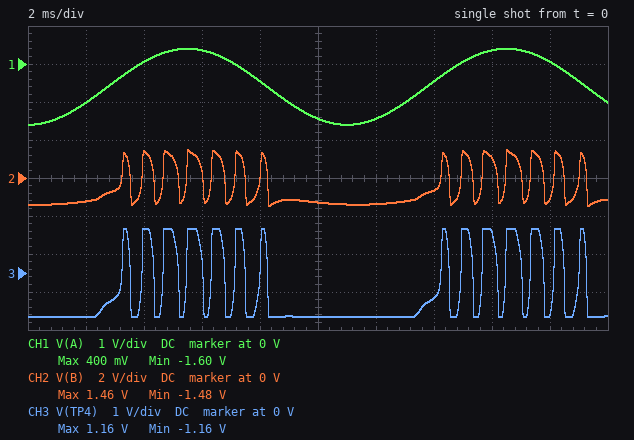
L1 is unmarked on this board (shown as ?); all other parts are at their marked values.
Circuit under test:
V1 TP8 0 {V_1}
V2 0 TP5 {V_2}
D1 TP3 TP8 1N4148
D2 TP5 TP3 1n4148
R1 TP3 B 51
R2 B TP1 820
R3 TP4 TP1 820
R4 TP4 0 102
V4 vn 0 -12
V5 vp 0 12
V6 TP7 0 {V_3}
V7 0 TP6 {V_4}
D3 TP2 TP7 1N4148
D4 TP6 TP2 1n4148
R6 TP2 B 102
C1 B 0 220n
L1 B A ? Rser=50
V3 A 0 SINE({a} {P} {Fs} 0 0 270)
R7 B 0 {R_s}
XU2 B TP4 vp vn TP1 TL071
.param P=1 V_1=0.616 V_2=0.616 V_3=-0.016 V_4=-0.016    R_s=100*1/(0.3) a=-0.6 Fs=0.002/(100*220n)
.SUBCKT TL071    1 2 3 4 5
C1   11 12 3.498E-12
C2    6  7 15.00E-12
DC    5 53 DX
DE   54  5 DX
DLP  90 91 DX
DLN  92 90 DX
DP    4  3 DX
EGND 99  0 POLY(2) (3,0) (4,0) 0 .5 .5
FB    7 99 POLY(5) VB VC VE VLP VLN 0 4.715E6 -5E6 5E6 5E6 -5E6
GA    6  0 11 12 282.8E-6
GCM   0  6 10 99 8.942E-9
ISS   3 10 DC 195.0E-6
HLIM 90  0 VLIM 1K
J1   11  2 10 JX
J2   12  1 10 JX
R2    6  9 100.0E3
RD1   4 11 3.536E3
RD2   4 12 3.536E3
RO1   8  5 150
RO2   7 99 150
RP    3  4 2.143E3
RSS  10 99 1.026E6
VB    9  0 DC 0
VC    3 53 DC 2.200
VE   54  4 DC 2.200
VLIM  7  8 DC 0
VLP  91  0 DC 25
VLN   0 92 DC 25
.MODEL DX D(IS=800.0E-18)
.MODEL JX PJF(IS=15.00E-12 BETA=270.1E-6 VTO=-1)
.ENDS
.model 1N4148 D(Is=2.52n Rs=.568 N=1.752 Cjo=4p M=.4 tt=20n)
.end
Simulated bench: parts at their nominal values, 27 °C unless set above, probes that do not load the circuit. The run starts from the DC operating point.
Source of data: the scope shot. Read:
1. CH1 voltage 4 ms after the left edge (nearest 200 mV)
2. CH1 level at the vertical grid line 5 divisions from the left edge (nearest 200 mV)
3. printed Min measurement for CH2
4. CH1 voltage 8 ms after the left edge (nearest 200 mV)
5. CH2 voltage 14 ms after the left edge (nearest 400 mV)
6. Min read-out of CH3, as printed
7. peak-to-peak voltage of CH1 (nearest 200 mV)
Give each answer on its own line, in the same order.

0 V
-1.4 V
-1.48 V
-400 mV
-800 mV
-1.16 V
2.0 V
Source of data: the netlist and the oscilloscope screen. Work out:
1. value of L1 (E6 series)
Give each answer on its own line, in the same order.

33 mH
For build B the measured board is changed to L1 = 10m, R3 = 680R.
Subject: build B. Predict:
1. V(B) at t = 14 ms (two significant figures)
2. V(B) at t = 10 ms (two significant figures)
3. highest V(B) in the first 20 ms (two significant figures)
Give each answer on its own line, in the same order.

-590 mV
-1.3 V
1.4 V
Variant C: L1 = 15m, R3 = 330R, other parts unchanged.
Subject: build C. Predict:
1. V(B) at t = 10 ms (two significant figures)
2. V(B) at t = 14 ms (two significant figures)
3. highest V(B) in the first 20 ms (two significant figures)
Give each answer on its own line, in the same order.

-1.2 V
-500 mV
430 mV
